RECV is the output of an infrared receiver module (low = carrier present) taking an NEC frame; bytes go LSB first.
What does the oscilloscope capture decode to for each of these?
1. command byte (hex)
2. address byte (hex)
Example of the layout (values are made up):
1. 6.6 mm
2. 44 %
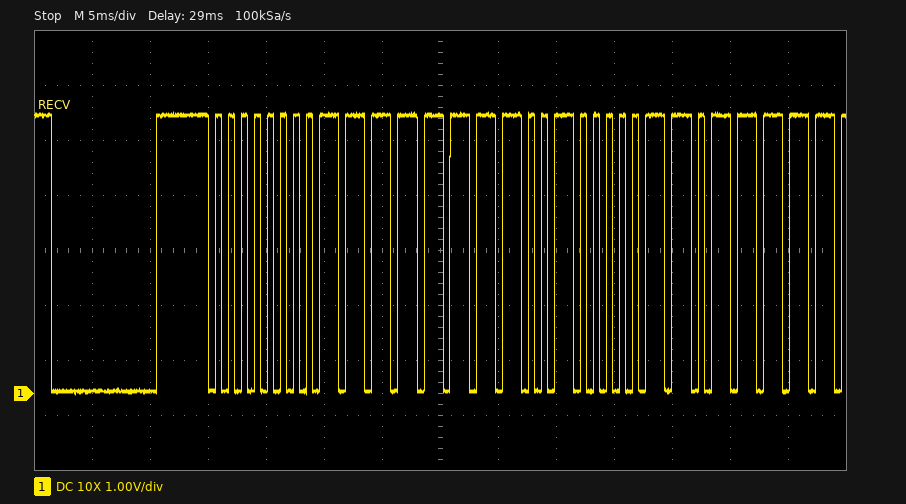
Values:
1. 0x04
2. 0x00
